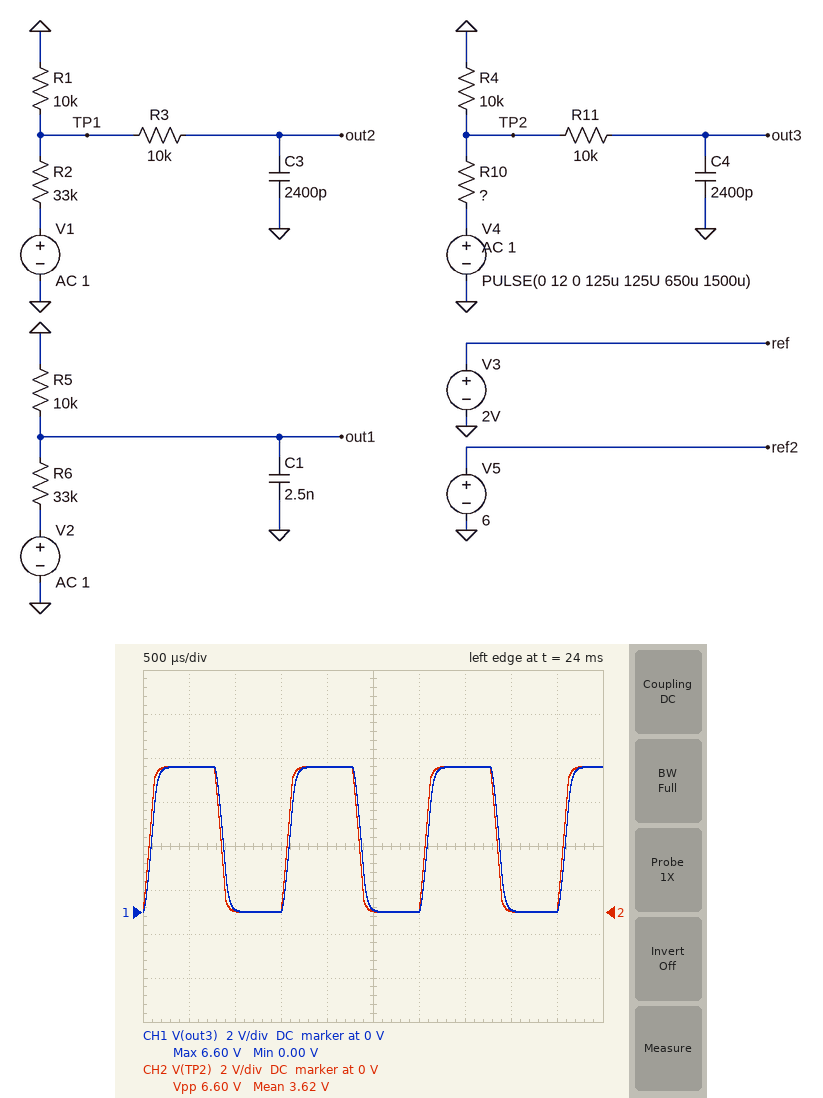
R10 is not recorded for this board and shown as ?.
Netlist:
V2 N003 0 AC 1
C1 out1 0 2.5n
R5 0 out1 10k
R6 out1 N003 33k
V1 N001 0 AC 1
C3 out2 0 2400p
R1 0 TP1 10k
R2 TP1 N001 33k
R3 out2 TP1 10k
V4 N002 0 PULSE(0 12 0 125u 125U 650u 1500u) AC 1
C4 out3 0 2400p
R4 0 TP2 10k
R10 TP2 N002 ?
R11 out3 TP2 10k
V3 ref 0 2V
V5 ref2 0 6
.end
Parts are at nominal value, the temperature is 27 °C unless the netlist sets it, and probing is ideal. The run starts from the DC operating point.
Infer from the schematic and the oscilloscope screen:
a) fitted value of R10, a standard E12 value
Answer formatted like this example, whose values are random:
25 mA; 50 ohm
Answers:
8.2 kΩ
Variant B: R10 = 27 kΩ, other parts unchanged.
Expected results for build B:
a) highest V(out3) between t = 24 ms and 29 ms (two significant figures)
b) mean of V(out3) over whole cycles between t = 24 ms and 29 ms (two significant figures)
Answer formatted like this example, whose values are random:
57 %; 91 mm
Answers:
3.2 V; 1.7 V
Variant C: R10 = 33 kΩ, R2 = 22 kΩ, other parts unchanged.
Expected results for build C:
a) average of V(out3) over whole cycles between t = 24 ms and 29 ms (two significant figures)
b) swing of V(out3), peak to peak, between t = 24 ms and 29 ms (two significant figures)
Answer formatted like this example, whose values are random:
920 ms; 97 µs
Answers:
1.4 V; 2.8 V
